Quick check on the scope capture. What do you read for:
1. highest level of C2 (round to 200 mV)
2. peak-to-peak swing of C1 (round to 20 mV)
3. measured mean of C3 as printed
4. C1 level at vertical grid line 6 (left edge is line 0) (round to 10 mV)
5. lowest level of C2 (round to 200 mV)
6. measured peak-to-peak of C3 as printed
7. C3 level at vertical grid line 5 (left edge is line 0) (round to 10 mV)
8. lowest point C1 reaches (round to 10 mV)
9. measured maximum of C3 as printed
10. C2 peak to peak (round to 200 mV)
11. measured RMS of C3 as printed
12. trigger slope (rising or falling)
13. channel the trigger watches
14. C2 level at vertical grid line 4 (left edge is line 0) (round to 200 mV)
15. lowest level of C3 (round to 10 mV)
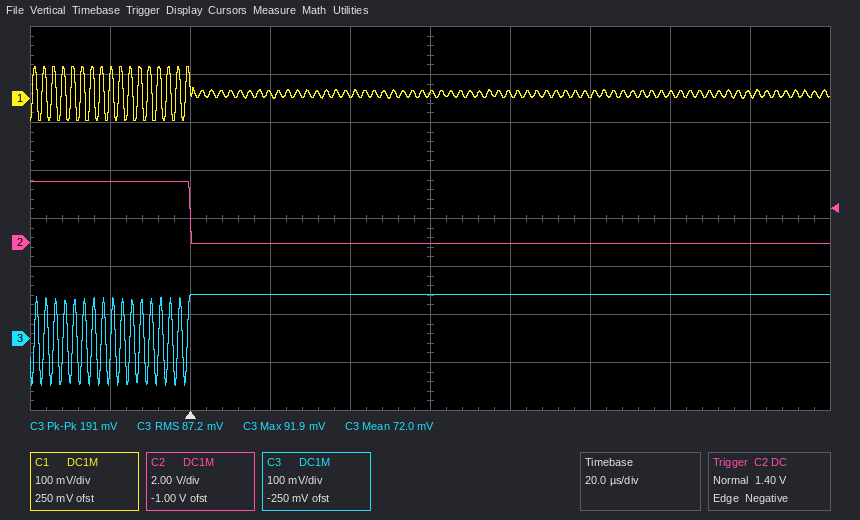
2.6 V
120 mV
72.0 mV
10 mV
0.0 V
191 mV
90 mV
-50 mV
91.9 mV
2.6 V
87.2 mV
falling
C2
0.0 V
-100 mV
